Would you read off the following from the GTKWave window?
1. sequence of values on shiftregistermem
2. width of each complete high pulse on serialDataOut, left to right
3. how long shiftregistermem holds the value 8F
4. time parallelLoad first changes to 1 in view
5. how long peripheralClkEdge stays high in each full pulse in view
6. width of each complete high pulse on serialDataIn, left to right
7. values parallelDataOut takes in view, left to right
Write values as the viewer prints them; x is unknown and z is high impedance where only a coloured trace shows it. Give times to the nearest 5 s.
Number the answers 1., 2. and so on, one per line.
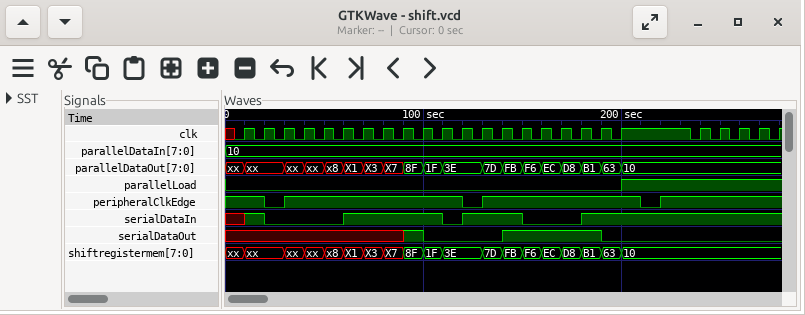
1. xx, xx, xx, xx, x8, X1, X3, X7, 8F, 1F, 3E, 7D, FB, F6, EC, D8, B1, 63, 10
2. 50 s
3. 10 s
4. 200 s
5. 90 s, 80 s
6. 50 s, 30 s
7. xx, xx, xx, xx, x8, X1, X3, X7, 8F, 1F, 3E, 7D, FB, F6, EC, D8, B1, 63, 10
